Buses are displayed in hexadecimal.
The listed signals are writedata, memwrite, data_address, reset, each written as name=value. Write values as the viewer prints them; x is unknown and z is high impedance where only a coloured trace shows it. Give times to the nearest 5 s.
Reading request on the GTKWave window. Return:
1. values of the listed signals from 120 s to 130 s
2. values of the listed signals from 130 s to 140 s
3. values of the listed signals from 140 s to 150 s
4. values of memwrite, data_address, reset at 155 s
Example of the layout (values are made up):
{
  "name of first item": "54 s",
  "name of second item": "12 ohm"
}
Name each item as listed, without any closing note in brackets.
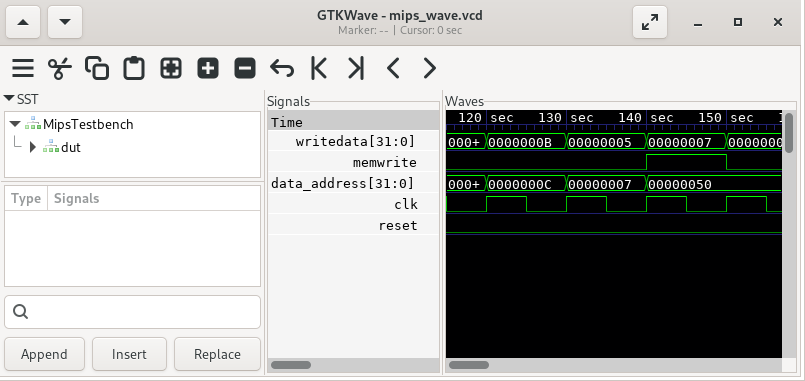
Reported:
{
  "values of the listed signals from 120 s to 130 s": "writedata=0000000B, memwrite=0, data_address=0000000C, reset=0",
  "values of the listed signals from 130 s to 140 s": "writedata=00000005, memwrite=0, data_address=00000007, reset=0",
  "values of the listed signals from 140 s to 150 s": "writedata=00000007, memwrite=1, data_address=00000050, reset=0",
  "values of memwrite, data_address, reset at 155 s": "memwrite=0, data_address=00000050, reset=0"
}
